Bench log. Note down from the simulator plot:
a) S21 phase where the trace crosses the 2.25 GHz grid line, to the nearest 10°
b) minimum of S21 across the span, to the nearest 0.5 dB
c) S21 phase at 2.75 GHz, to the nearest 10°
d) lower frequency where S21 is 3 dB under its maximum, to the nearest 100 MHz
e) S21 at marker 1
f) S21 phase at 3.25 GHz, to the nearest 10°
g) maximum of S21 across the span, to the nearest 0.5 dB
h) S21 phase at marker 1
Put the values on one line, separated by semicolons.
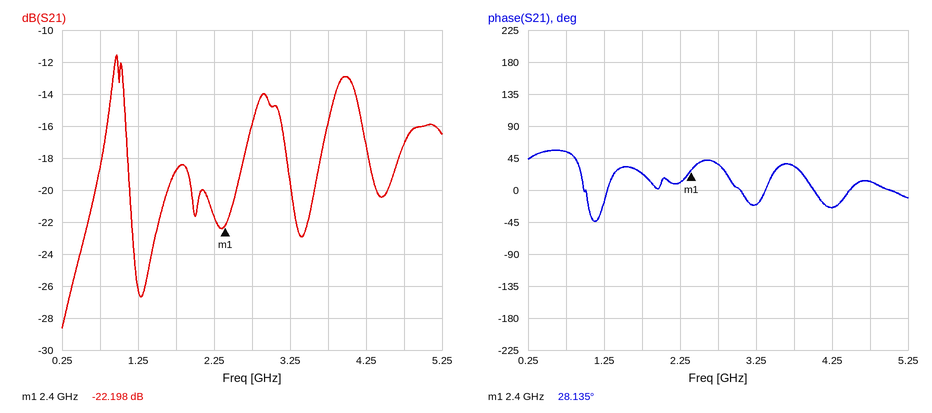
10°; -28.5 dB; 40°; 900 MHz; -22.198 dB; -20°; -11.5 dB; 28.135°
